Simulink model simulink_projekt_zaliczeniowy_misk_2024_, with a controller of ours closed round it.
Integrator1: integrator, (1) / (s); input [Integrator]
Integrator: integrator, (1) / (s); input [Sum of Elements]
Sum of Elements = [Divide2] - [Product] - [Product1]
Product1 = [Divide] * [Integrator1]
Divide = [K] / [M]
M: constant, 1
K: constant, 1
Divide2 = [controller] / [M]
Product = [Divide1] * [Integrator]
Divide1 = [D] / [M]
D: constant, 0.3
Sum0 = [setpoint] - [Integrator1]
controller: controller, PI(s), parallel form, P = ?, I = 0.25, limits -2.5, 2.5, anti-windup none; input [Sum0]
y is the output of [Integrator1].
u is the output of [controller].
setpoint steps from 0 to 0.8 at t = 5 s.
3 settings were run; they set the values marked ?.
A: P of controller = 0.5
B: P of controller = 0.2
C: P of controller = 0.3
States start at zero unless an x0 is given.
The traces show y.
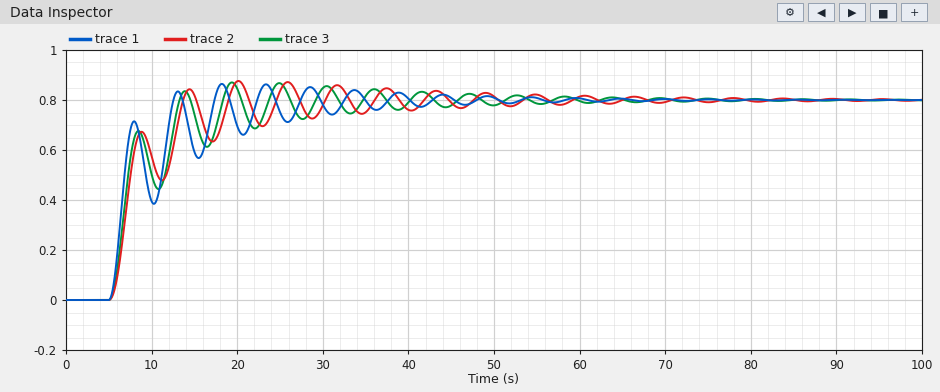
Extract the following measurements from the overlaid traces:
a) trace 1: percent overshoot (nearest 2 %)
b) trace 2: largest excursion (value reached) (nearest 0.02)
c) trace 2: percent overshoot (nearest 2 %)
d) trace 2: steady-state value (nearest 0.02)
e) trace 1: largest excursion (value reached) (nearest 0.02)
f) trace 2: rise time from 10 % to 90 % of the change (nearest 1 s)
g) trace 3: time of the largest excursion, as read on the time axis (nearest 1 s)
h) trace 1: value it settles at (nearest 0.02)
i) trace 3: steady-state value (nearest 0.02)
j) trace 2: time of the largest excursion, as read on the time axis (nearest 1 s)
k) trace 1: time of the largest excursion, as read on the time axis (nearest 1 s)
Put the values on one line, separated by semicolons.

8 %; 0.88; 10 %; 0.80; 0.86; 7 s; 19 s; 0.80; 0.80; 20 s; 18 s
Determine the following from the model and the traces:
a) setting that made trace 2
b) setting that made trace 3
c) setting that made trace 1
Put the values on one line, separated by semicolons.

B; C; A
